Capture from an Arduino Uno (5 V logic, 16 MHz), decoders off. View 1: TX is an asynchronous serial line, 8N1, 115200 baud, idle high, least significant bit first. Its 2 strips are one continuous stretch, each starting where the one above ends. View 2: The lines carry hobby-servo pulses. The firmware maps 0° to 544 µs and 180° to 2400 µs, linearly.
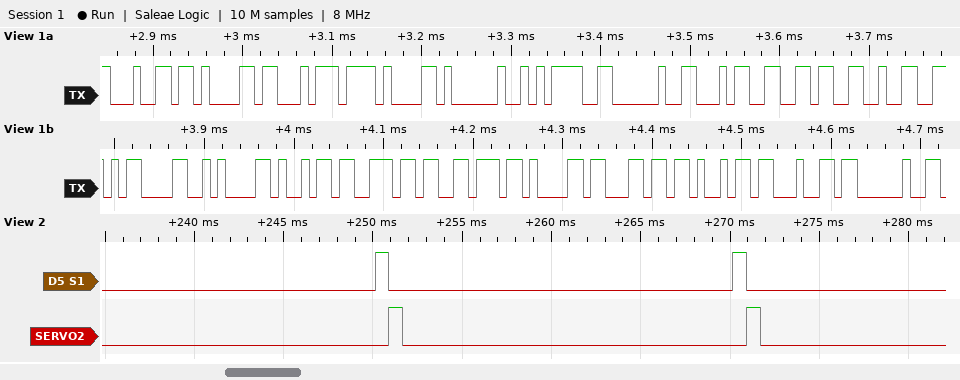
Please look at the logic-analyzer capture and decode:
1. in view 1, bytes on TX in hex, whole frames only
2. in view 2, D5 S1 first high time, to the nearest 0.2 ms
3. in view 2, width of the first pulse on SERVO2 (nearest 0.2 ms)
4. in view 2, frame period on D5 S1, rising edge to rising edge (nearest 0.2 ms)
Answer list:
64 61 74 61 20 3D 20 34 36 32 0D 0A 69 6E 76 61 6C 69 64 20
0.8 ms
0.8 ms
20.0 ms
